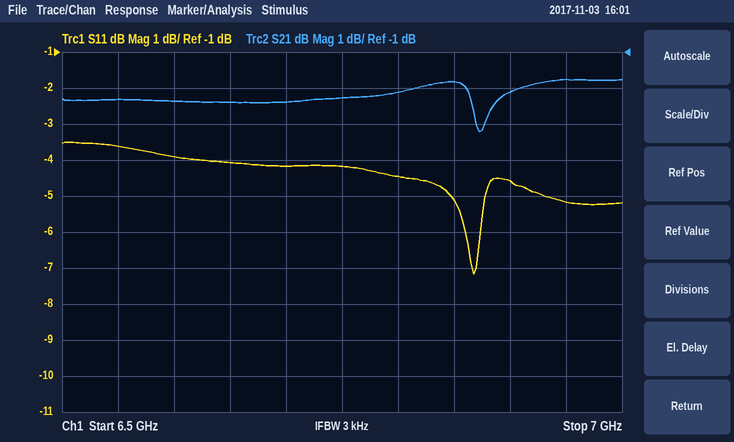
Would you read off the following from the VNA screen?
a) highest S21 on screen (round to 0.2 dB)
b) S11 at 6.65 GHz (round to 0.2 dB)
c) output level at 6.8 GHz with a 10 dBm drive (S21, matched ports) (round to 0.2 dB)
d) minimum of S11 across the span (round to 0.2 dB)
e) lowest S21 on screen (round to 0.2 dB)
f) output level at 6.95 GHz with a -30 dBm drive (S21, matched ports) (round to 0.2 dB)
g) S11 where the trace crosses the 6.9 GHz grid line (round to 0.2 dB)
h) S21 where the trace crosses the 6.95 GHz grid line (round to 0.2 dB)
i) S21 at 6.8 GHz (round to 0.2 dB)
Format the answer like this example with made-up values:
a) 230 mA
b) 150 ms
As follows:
a) -1.8 dB
b) -4.0 dB
c) 7.8 dBm
d) -7.2 dB
e) -3.2 dB
f) -31.8 dBm
g) -4.6 dB
h) -1.8 dB
i) -2.2 dB
